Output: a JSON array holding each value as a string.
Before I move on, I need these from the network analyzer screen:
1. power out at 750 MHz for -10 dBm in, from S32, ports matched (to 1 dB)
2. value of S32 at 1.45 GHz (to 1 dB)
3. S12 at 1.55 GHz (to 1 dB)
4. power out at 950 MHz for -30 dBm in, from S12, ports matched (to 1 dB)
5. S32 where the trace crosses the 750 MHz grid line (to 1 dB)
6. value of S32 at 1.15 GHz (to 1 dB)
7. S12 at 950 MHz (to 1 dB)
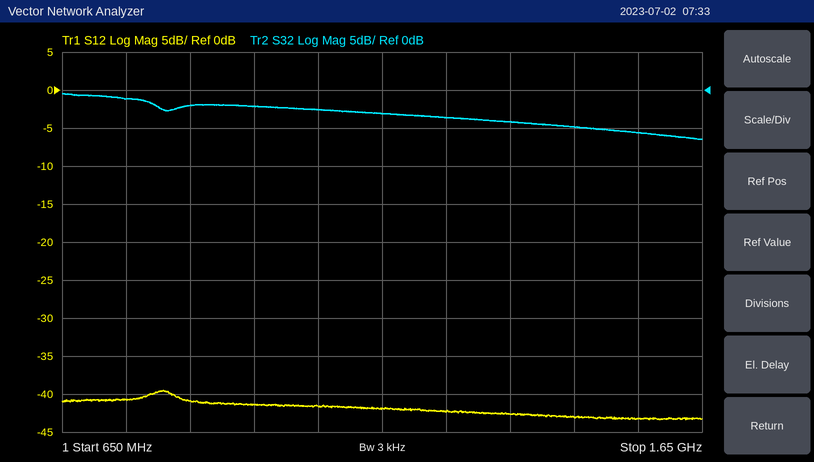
["-11 dBm", "-5 dB", "-43 dB", "-71 dBm", "-1 dB", "-3 dB", "-41 dB"]
